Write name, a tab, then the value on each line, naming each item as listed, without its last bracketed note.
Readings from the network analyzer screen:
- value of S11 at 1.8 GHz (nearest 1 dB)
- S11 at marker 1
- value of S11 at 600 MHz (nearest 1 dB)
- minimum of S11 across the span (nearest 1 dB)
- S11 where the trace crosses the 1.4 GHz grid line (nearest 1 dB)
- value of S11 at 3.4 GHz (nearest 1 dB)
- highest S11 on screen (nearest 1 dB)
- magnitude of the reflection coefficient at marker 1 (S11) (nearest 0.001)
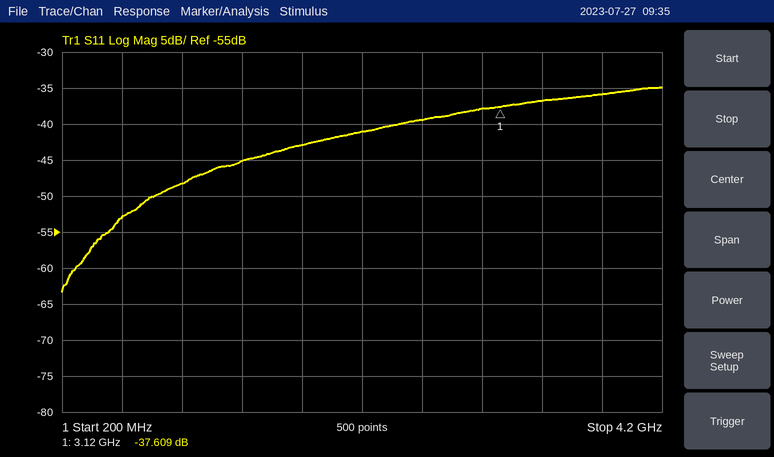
value of S11 at 1.8 GHz	-43 dB
S11 at marker 1	-37.609 dB
value of S11 at 600 MHz	-53 dB
minimum of S11 across the span	-63 dB
S11 where the trace crosses the 1.4 GHz grid line	-45 dB
value of S11 at 3.4 GHz	-37 dB
highest S11 on screen	-35 dB
magnitude of the reflection coefficient at marker 1 (S11)	0.013
